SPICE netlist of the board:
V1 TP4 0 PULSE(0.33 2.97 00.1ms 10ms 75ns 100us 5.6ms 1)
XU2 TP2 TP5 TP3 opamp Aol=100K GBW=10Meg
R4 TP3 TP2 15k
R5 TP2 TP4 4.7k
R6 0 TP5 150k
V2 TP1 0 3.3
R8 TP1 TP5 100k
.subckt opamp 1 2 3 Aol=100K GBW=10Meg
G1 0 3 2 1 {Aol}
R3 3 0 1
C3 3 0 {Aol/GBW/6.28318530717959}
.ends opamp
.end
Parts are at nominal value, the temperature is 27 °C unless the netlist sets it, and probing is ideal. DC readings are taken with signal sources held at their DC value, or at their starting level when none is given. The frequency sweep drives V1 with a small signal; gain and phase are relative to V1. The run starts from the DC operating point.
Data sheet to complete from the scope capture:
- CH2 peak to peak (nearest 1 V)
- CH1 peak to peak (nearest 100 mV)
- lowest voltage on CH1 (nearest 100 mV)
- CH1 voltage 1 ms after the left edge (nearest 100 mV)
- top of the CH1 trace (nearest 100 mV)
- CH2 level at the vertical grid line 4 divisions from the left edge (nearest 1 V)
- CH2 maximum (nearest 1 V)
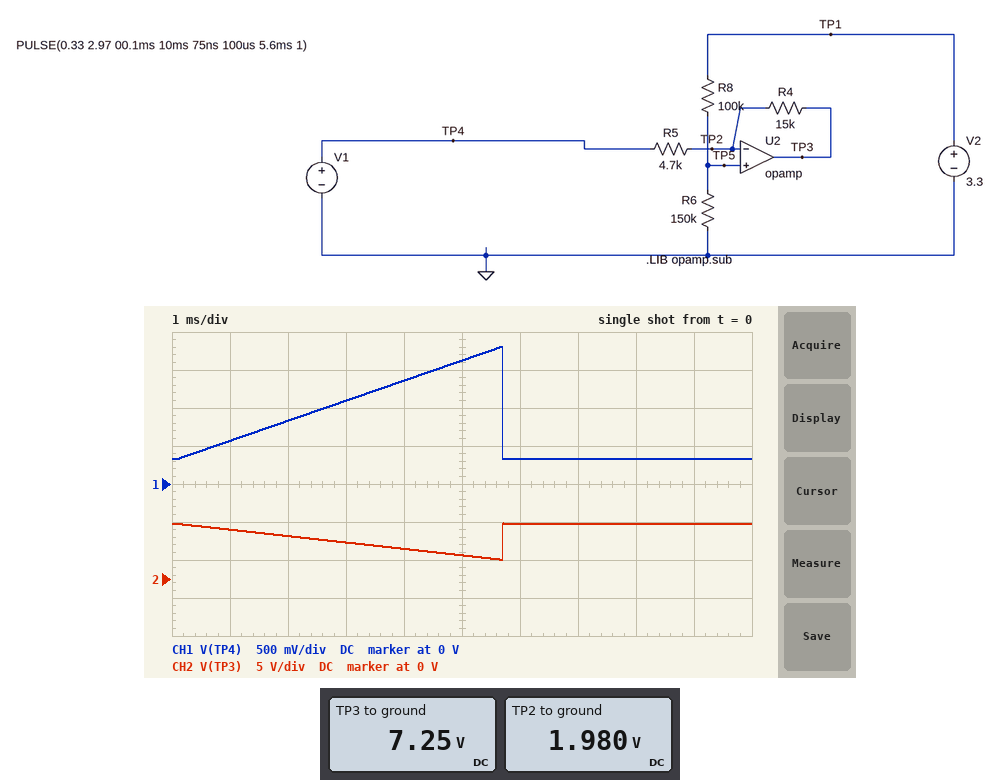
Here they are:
5 V
1.5 V
300 mV
600 mV
1.8 V
4 V
7 V
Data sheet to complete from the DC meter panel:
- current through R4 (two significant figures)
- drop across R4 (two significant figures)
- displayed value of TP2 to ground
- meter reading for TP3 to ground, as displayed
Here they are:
350 µA
5.3 V
1.980 V
7.25 V
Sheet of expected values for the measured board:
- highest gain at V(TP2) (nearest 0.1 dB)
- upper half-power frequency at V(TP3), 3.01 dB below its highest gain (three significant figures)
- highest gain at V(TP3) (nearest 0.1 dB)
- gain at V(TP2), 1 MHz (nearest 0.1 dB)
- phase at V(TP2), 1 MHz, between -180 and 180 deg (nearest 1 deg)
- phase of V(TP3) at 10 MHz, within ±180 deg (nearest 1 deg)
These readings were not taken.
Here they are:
-2.4 dB
2.39 MHz
10.1 dB
-10.6 dB
67 deg
103 deg
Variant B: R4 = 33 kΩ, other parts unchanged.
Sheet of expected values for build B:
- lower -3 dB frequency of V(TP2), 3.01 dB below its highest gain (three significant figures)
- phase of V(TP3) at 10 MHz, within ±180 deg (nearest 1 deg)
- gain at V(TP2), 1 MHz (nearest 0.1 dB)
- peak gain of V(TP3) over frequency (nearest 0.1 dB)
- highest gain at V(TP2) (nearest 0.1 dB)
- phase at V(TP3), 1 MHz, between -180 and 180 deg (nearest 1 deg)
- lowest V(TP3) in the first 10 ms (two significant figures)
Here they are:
1.25 MHz
97 deg
-5.2 dB
16.9 dB
-1.2 dB
141 deg
3.2 V
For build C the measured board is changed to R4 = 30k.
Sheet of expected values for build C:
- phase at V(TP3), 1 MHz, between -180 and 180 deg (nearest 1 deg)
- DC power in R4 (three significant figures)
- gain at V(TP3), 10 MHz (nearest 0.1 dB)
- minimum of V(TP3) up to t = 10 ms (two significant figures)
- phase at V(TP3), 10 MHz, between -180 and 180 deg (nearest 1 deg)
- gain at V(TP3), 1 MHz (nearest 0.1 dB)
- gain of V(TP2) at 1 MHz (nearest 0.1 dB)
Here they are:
144 deg
3.70 mW
-1.3 dB
3.1 V
98 deg
14.2 dB
-5.8 dB
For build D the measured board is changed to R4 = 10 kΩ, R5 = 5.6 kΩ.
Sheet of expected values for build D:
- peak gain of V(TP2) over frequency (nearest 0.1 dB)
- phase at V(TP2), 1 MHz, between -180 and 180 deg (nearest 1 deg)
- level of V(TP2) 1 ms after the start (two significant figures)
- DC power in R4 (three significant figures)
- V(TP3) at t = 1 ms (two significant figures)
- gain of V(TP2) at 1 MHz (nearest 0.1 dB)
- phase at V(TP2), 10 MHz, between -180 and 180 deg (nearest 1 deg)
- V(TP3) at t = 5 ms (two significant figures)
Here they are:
-3.9 dB
74 deg
2.0 V
868 µW
4.5 V
-15.3 dB
20 deg
2.6 V
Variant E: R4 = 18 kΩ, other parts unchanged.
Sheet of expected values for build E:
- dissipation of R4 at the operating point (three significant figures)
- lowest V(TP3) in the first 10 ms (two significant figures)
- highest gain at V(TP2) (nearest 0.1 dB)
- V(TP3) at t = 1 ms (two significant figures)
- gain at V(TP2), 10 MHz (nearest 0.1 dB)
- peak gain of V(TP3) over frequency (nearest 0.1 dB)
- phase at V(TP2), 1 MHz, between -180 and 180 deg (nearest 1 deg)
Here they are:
2.22 mW
2.6 V
-2.0 dB
7.4 V
-2.2 dB
11.7 dB
64 deg
